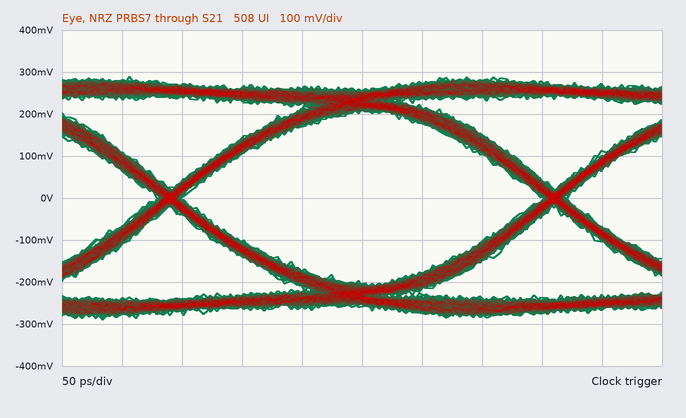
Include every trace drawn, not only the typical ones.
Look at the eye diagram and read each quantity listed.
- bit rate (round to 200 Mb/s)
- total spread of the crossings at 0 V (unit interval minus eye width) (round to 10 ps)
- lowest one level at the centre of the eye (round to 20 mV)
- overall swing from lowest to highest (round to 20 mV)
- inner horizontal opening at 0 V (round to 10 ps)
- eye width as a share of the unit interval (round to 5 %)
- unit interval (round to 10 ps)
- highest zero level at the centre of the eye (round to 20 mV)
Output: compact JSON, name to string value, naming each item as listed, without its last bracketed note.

{"bit rate": "3.2 Gb/s", "total spread of the crossings at 0 V (unit interval minus eye width)": "20 ps", "lowest one level at the centre of the eye": "200 mV", "overall swing from lowest to highest": "580 mV", "inner horizontal opening at 0 V": "300 ps", "eye width as a share of the unit interval": "95 %", "unit interval": "320 ps", "highest zero level at the centre of the eye": "-200 mV"}
